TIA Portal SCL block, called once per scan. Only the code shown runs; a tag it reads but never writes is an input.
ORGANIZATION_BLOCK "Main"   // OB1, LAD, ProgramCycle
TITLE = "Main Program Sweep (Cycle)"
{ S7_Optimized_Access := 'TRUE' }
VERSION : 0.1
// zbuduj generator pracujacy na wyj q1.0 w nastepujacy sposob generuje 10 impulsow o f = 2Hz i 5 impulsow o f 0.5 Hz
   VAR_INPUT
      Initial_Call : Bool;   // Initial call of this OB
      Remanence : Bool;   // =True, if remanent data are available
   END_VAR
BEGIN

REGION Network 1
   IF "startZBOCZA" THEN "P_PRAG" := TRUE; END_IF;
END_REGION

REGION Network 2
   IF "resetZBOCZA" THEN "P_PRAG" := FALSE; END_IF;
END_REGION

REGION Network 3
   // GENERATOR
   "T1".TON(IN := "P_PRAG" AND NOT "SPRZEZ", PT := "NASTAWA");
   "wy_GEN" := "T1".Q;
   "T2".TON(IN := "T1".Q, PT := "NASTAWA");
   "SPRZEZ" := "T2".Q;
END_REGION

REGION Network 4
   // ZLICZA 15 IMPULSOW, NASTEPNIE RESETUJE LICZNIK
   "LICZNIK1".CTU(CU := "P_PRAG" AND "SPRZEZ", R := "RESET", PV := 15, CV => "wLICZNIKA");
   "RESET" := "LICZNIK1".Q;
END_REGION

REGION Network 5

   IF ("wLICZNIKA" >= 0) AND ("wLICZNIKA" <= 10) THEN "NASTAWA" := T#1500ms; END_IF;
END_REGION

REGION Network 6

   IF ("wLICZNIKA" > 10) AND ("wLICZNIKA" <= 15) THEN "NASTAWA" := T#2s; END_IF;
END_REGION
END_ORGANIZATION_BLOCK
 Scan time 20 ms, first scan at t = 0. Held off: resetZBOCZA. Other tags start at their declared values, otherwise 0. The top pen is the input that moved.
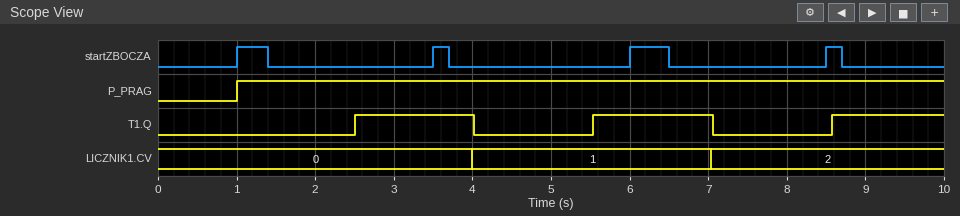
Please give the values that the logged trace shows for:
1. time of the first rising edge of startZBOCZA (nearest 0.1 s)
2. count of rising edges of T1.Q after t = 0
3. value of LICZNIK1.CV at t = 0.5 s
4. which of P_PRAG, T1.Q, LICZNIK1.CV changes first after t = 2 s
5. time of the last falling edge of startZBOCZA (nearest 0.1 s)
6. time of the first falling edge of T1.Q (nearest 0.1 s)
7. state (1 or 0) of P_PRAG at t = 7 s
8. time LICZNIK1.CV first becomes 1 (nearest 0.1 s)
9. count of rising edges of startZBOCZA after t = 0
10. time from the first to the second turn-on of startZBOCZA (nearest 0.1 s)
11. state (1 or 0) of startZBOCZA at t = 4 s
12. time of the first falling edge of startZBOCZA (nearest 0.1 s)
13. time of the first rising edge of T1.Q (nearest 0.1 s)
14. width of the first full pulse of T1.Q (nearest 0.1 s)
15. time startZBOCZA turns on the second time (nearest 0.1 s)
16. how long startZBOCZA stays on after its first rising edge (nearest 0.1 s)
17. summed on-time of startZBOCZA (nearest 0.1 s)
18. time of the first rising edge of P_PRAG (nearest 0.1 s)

1.0 s
3
0
T1.Q
8.7 s
4.0 s
1
4.0 s
4
2.5 s
0
1.4 s
2.5 s
1.5 s
3.5 s
0.4 s
1.3 s
1.0 s
